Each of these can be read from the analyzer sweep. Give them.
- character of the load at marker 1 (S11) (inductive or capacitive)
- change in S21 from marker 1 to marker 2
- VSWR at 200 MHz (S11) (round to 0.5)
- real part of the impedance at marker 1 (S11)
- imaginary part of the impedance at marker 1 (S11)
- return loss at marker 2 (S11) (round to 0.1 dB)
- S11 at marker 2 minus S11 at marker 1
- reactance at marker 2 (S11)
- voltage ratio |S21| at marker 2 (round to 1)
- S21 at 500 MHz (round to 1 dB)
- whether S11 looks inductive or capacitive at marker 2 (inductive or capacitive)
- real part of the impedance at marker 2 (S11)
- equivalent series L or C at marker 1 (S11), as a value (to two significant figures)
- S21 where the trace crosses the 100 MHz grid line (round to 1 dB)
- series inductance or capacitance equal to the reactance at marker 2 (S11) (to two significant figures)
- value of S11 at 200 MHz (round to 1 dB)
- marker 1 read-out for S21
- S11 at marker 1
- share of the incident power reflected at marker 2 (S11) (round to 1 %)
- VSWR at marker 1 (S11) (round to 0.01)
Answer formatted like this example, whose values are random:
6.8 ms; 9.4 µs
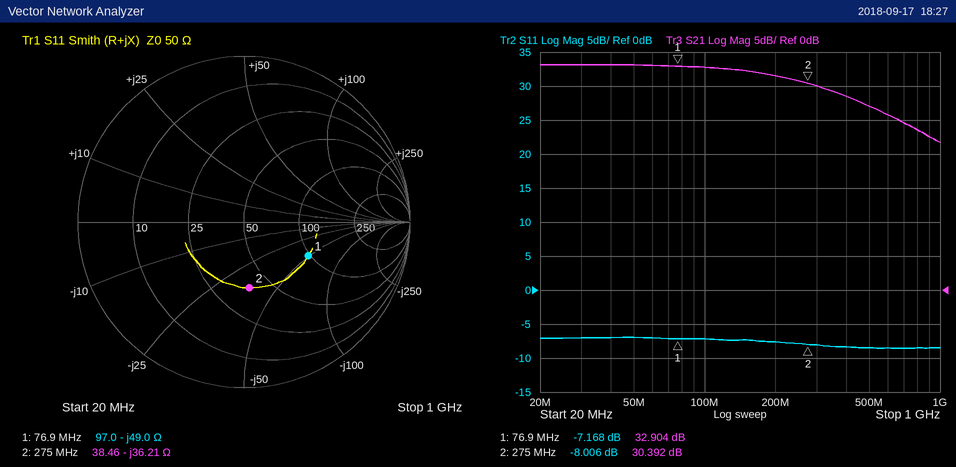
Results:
capacitive; -2.512 dB; 2.5; 97.0 Ω; -49.0 Ω; 8.0 dB; -0.838 dB; -36.21 Ω; 33; 27 dB; capacitive; 38.46 Ω; 42 pF; 33 dB; 16 pF; -8 dB; 32.904 dB; -7.168 dB; 16 %; 2.56
